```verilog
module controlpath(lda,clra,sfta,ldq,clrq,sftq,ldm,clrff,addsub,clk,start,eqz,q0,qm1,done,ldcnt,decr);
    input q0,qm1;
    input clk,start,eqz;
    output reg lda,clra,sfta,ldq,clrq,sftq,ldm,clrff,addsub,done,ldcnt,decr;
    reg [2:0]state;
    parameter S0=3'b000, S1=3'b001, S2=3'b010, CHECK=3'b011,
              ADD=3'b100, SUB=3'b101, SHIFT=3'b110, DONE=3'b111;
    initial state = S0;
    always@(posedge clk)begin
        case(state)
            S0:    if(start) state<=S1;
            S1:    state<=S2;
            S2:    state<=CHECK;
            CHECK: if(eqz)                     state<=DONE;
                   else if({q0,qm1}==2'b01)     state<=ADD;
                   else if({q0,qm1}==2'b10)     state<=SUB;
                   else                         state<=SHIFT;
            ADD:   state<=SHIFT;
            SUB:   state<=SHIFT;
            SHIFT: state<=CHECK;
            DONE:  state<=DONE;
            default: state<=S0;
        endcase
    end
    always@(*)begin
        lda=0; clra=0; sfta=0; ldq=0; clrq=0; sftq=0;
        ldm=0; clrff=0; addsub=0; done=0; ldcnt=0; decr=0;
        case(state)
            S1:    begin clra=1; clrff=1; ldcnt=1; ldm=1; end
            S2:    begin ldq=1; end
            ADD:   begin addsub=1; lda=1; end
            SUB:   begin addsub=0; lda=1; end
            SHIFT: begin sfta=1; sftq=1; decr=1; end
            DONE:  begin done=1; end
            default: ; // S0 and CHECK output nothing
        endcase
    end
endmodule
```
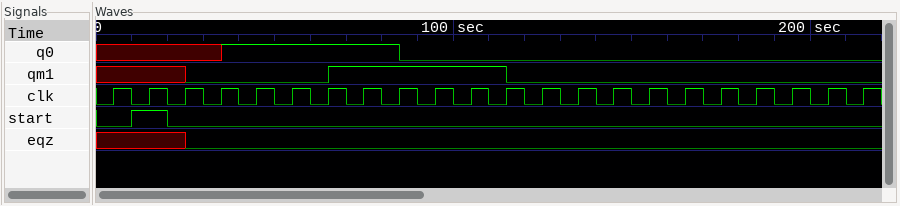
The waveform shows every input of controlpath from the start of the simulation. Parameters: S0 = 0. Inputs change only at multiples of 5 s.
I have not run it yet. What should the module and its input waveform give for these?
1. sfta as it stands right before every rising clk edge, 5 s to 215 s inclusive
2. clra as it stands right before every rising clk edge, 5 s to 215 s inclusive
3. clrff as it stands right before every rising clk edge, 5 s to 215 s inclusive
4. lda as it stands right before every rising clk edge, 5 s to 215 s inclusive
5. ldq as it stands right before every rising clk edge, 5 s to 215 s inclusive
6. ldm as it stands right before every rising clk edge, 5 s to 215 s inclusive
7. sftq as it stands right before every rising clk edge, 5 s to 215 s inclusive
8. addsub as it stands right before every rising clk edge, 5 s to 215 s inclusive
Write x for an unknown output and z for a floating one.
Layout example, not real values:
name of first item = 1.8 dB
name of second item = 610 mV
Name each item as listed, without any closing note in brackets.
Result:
sfta as it stands right before every rising clk edge, 5 s to 215 s inclusive = 0 0 0 0 0 0 1 0 1 0 0 1 0 1 0 1 0 1 0 1 0 1
clra as it stands right before every rising clk edge, 5 s to 215 s inclusive = 0 0 1 0 0 0 0 0 0 0 0 0 0 0 0 0 0 0 0 0 0 0
clrff as it stands right before every rising clk edge, 5 s to 215 s inclusive = 0 0 1 0 0 0 0 0 0 0 0 0 0 0 0 0 0 0 0 0 0 0
lda as it stands right before every rising clk edge, 5 s to 215 s inclusive = 0 0 0 0 0 1 0 0 0 0 1 0 0 0 0 0 0 0 0 0 0 0
ldq as it stands right before every rising clk edge, 5 s to 215 s inclusive = 0 0 0 1 0 0 0 0 0 0 0 0 0 0 0 0 0 0 0 0 0 0
ldm as it stands right before every rising clk edge, 5 s to 215 s inclusive = 0 0 1 0 0 0 0 0 0 0 0 0 0 0 0 0 0 0 0 0 0 0
sftq as it stands right before every rising clk edge, 5 s to 215 s inclusive = 0 0 0 0 0 0 1 0 1 0 0 1 0 1 0 1 0 1 0 1 0 1
addsub as it stands right before every rising clk edge, 5 s to 215 s inclusive = 0 0 0 0 0 0 0 0 0 0 1 0 0 0 0 0 0 0 0 0 0 0
